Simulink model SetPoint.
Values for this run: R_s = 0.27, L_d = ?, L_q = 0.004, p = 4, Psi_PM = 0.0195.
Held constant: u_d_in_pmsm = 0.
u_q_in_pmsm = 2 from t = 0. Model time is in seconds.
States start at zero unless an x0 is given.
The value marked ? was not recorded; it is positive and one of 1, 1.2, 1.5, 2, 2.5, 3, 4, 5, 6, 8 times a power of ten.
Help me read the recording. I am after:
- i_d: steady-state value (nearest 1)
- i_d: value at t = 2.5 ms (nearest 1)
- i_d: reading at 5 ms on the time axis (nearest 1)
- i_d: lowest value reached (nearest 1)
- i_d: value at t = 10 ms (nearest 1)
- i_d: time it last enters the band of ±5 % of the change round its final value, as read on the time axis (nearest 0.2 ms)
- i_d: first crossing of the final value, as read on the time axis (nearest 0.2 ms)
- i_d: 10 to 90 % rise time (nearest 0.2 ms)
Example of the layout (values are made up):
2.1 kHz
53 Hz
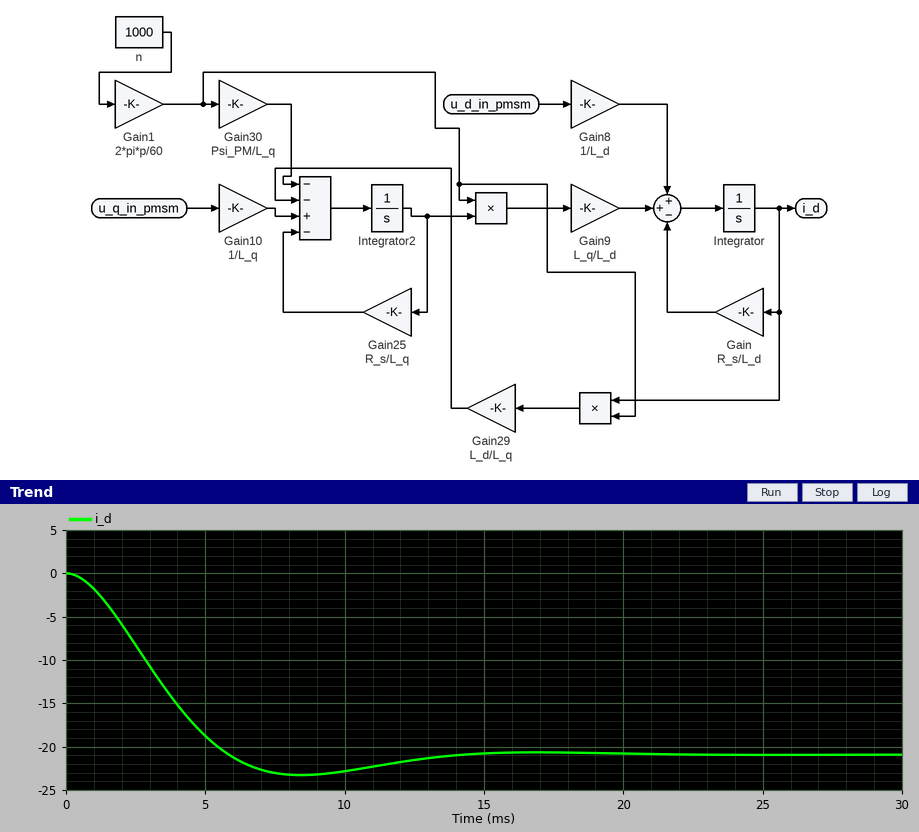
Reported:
-21
-8
-19
-23
-23
11.6 ms
5.8 ms
4.0 ms
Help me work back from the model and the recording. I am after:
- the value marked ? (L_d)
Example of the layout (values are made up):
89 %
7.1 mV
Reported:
0.0006
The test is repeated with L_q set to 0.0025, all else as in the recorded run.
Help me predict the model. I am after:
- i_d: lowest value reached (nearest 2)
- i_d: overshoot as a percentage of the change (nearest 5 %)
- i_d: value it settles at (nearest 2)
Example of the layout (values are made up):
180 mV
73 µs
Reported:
-22
10 %
-20
